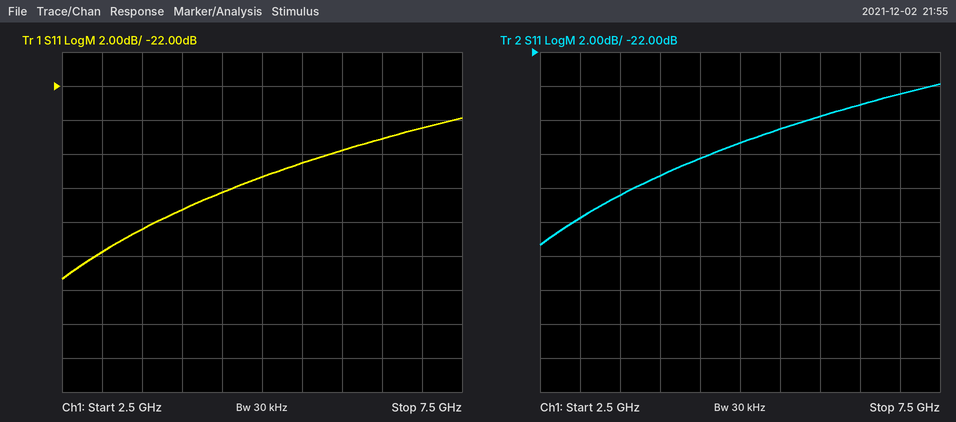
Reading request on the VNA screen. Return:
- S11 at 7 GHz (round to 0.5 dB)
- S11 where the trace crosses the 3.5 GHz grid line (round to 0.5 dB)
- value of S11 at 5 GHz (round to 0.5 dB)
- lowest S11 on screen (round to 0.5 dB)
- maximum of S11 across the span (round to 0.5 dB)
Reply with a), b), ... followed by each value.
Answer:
a) -24.5 dB
b) -30.5 dB
c) -27.5 dB
d) -33.5 dB
e) -24.0 dB
